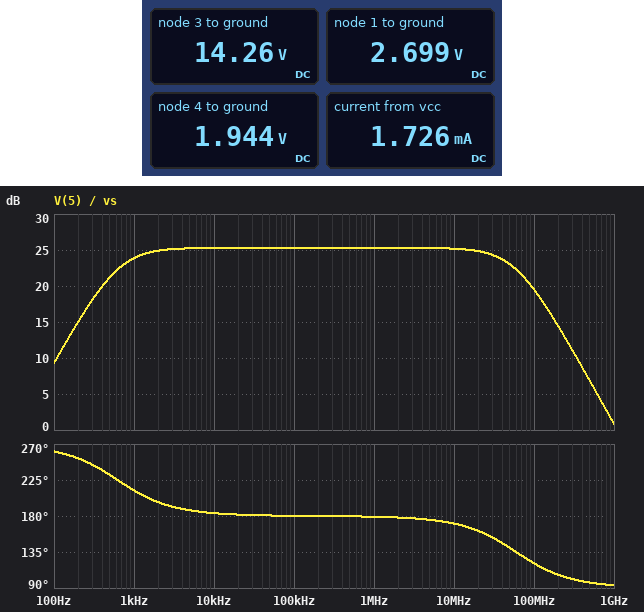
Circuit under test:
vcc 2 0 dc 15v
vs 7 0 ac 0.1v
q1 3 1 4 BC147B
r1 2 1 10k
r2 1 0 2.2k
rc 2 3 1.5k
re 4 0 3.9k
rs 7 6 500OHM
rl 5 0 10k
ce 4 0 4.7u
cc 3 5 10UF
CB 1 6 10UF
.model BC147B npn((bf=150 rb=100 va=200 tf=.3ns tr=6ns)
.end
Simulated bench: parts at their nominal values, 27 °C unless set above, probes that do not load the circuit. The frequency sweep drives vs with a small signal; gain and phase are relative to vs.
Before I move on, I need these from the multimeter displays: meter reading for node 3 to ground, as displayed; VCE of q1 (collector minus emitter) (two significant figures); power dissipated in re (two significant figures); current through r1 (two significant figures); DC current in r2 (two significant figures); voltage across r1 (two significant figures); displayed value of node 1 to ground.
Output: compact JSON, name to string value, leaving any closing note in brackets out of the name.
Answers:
{"meter reading for node 3 to ground, as displayed": "14.26 V", "VCE of q1 (collector minus emitter)": "12 V", "power dissipated in re": "970 µW", "current through r1": "1.2 mA", "DC current in r2": "1.2 mA", "voltage across r1": "12 V", "displayed value of node 1 to ground": "2.699 V"}
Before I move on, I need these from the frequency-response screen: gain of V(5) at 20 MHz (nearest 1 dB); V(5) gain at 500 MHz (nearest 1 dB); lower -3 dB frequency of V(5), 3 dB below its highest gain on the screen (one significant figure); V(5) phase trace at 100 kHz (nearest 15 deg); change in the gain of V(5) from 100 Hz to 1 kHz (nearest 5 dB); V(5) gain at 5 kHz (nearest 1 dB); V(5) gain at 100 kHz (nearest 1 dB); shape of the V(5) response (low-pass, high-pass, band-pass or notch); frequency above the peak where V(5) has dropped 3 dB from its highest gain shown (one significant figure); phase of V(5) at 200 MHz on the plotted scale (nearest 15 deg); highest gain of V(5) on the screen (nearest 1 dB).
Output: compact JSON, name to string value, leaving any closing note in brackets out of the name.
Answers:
{"gain of V(5) at 20 MHz": "25 dB", "V(5) gain at 500 MHz": "7 dB", "lower -3 dB frequency of V(5), 3 dB below its highest gain on the screen": "600 Hz", "V(5) phase trace at 100 kHz": "180 deg", "change in the gain of V(5) from 100 Hz to 1 kHz": "15 dB", "V(5) gain at 5 kHz": "25 dB", "V(5) gain at 100 kHz": "25 dB", "shape of the V(5) response": "band-pass", "frequency above the peak where V(5) has dropped 3 dB from its highest gain shown": "60 MHz", "phase of V(5) at 200 MHz on the plotted scale": "105 deg", "highest gain of V(5) on the screen": "25 dB"}
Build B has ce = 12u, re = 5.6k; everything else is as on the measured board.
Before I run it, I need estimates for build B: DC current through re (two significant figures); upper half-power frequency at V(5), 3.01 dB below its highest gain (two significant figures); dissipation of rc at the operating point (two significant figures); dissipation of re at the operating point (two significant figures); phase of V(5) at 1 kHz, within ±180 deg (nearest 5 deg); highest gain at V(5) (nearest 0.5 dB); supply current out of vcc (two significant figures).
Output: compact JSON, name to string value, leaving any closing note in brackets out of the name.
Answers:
{"DC current through re": "350 µA", "upper half-power frequency at V(5), 3.01 dB below its highest gain": "84 MHz", "dissipation of rc at the operating point": "180 µW", "dissipation of re at the operating point": "680 µW", "phase of V(5) at 1 kHz, within ±180 deg": "-170 deg", "highest gain at V(5)": "22.5 dB", "supply current out of vcc": "1.6 mA"}
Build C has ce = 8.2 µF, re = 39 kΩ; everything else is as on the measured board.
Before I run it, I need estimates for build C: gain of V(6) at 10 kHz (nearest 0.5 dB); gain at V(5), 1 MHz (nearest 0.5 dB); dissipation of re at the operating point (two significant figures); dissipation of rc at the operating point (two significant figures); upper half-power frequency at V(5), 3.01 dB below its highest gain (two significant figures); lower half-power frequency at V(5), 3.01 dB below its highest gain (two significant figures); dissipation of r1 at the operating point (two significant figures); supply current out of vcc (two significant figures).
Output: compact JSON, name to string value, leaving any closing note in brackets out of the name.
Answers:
{"gain of V(6) at 10 kHz": "-2.0 dB", "gain at V(5), 1 MHz": "6.0 dB", "dissipation of re at the operating point": "100 µW", "dissipation of rc at the operating point": "3.9 µW", "upper half-power frequency at V(5), 3.01 dB below its highest gain": "550 MHz", "lower half-power frequency at V(5), 3.01 dB below its highest gain": "40 Hz", "dissipation of r1 at the operating point": "15 mW", "supply current out of vcc": "1.3 mA"}
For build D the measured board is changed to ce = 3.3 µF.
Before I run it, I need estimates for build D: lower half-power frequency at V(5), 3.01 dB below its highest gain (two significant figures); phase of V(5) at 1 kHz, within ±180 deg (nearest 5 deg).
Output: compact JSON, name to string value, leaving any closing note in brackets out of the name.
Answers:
{"lower half-power frequency at V(5), 3.01 dB below its highest gain": "890 Hz", "phase of V(5) at 1 kHz, within ±180 deg": "-140 deg"}
